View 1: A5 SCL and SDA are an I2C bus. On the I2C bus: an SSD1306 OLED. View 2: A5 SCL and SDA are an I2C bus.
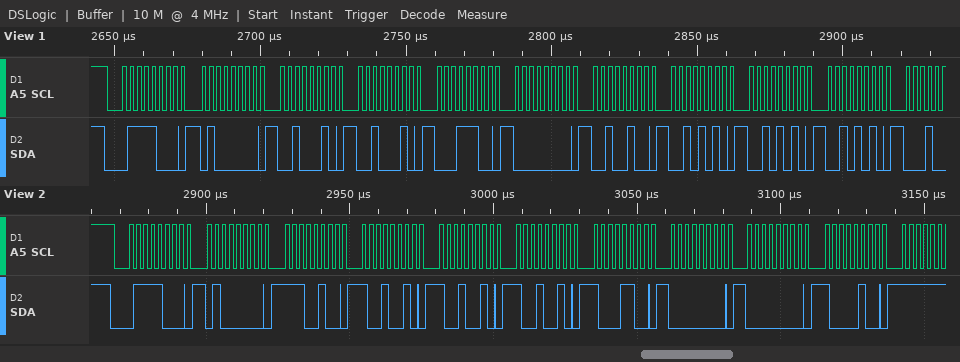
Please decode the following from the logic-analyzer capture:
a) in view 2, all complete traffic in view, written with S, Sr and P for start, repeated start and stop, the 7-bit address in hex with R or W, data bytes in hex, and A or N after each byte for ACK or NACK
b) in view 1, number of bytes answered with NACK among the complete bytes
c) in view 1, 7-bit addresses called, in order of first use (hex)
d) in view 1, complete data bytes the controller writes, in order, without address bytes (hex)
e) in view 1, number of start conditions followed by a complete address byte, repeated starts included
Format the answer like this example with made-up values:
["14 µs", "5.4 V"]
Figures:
["S 3CW A 40 A E4 A 92 A 92 A 92 A 8C A 00 A 00 A 84 A", "0", "0x3C", "40 22 22 1C 00 24 2A 2A 2A", "1"]
